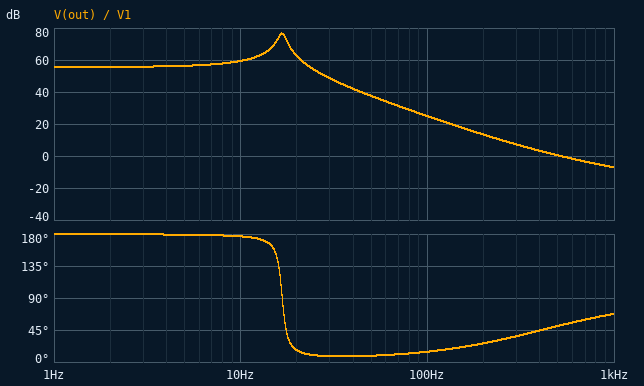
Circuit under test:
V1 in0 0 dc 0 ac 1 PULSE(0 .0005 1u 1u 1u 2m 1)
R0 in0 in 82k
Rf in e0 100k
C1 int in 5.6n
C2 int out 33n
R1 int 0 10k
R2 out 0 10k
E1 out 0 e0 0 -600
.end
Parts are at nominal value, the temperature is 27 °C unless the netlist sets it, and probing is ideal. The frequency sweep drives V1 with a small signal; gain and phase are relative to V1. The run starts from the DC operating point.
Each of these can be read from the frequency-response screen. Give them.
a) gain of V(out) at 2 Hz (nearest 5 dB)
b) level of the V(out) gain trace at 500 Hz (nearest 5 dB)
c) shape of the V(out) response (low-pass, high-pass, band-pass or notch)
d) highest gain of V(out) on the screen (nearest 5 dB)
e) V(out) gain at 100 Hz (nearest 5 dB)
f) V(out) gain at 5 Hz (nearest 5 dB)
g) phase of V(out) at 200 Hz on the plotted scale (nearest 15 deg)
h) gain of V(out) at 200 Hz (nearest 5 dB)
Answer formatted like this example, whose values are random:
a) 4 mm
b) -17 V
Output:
a) 55 dB
b) 0 dB
c) low-pass
d) 75 dB
e) 25 dB
f) 55 dB
g) 30 deg
h) 15 dB
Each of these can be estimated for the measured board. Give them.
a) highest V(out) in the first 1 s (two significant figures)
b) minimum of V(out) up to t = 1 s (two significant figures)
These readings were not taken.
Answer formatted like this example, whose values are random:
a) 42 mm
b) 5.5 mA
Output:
a) 51 mV
b) -59 mV
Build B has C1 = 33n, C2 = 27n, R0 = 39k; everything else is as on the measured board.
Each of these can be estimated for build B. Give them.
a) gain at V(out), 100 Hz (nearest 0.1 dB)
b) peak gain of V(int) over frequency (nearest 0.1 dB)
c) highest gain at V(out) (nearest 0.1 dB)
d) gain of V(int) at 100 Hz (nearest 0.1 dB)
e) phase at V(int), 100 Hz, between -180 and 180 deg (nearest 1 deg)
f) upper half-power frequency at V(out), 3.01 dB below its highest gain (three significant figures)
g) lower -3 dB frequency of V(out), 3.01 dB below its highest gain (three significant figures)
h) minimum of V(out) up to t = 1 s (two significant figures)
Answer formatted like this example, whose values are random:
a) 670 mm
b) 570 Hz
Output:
a) 17.9 dB
b) 38.7 dB
c) 73.3 dB
d) 1.9 dB
e) 91 deg
f) 11.7 Hz
g) 10.2 Hz
h) -38 mV
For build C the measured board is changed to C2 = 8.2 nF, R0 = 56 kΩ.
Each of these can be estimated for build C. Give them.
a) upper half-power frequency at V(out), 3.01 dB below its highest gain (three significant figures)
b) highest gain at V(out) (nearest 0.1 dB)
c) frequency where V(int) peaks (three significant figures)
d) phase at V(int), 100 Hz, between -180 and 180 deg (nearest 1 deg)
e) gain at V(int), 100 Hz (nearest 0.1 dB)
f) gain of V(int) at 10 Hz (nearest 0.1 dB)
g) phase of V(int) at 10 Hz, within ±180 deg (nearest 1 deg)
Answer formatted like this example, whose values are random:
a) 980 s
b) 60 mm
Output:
a) 42.6 Hz
b) 74.4 dB
c) 40.5 Hz
d) 93 deg
e) 15.6 dB
f) 10.3 dB
g) -92 deg
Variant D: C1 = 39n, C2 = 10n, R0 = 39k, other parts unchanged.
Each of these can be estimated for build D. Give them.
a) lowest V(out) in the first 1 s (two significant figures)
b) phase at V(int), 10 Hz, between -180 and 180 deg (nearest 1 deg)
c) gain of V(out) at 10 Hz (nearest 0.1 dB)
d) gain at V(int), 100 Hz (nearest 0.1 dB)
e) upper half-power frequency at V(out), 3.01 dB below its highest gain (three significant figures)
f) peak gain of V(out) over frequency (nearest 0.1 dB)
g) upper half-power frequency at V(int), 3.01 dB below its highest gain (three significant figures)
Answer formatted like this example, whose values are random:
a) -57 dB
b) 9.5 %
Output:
a) -54 mV
b) -101 deg
c) 59.3 dB
d) 0.6 dB
e) 18.1 Hz
f) 69.2 dB
g) 18.5 Hz
